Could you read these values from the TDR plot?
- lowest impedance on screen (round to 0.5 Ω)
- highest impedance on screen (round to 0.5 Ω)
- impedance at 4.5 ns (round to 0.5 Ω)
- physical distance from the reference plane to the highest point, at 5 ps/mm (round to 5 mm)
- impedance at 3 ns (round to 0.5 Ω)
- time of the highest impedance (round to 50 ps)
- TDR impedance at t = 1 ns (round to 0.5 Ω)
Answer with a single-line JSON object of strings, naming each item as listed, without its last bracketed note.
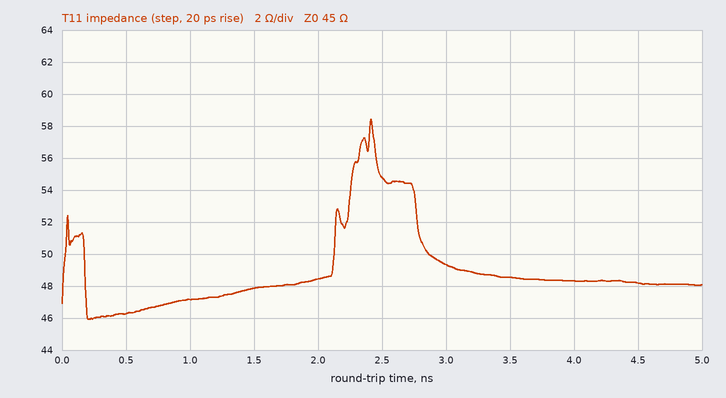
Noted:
{"lowest impedance on screen": "46.0 Ω", "highest impedance on screen": "58.5 Ω", "impedance at 4.5 ns": "48.0 Ω", "physical distance from the reference plane to the highest point, at 5 ps/mm": "240 mm", "impedance at 3 ns": "49.5 Ω", "time of the highest impedance": "2.40 ns", "TDR impedance at t = 1 ns": "47.0 Ω"}
